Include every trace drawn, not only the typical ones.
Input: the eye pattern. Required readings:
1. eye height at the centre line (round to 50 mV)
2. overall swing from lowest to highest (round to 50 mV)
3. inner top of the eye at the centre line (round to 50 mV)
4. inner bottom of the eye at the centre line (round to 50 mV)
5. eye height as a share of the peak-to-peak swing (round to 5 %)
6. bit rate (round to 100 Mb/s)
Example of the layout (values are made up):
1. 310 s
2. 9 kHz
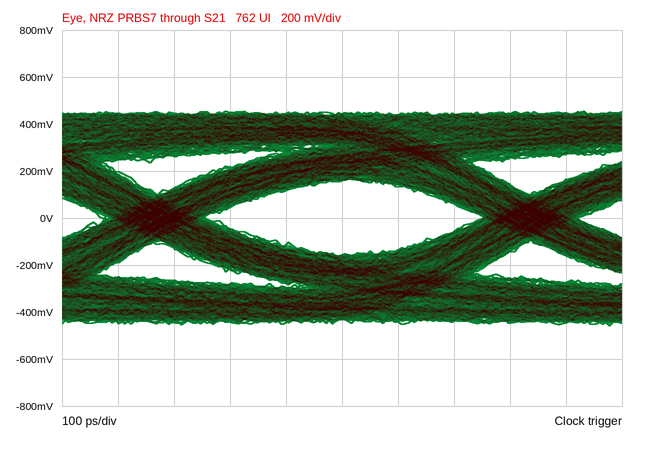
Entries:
1. 300 mV
2. 900 mV
3. 150 mV
4. -150 mV
5. 35 %
6. 1.5 Gb/s
